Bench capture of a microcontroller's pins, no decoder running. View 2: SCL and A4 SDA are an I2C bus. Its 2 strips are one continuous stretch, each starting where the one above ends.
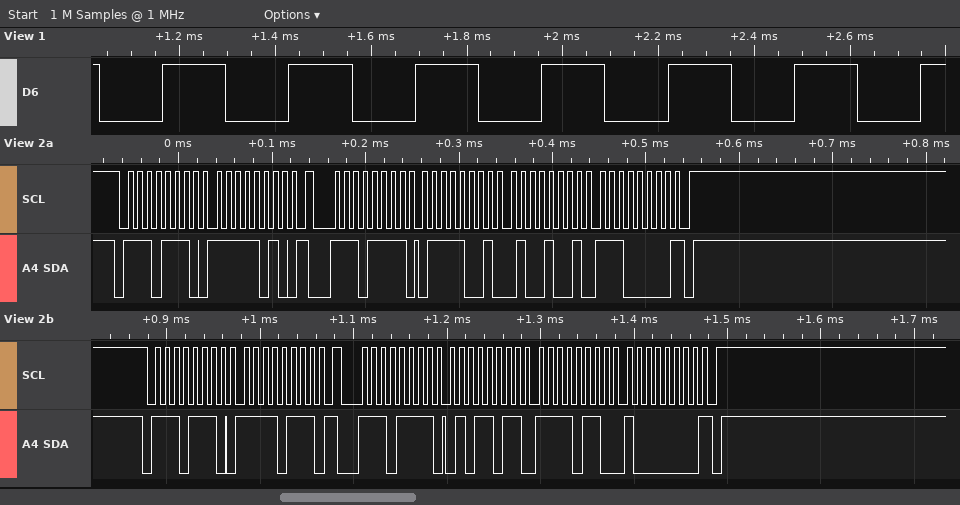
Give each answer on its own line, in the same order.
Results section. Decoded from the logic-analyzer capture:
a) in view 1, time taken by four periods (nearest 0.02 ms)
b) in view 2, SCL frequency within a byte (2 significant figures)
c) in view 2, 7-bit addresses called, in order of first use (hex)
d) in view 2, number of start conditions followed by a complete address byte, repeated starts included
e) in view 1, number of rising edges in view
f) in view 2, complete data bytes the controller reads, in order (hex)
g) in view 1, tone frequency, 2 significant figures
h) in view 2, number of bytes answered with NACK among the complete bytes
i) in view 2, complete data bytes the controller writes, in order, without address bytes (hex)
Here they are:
1.06 ms
100 kHz
0x77
4
7
79 49 E0 5B F6 80
3.8 kHz
2
FA F7
